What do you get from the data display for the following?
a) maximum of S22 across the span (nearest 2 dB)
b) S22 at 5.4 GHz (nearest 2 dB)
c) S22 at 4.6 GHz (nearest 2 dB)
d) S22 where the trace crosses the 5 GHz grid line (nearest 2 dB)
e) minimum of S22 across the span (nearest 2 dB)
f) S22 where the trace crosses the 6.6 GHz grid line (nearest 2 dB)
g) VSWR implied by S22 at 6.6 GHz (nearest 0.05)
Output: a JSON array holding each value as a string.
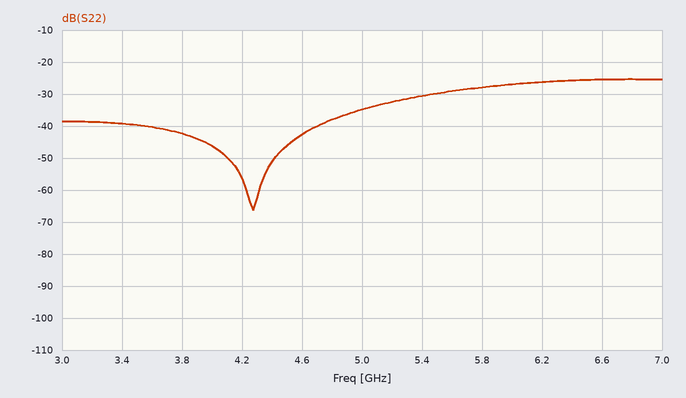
["-26 dB", "-30 dB", "-42 dB", "-34 dB", "-66 dB", "-26 dB", "1.10"]
